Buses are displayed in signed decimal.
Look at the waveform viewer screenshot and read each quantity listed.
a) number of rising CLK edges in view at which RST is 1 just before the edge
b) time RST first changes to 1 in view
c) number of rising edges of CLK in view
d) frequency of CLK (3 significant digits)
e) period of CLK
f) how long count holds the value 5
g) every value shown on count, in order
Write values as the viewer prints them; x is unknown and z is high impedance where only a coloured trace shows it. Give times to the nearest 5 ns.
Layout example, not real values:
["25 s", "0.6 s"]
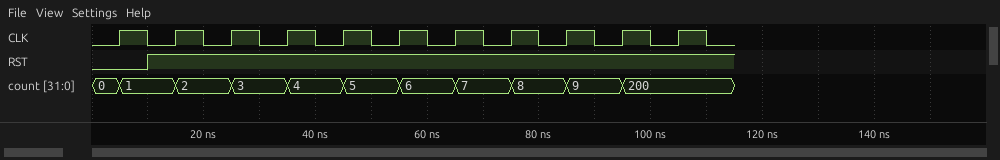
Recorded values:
["10", "10 ns", "11", "100 MHz", "10 ns", "10 ns", "0, 1, 2, 3, 4, 5, 6, 7, 8, 9, 200"]
